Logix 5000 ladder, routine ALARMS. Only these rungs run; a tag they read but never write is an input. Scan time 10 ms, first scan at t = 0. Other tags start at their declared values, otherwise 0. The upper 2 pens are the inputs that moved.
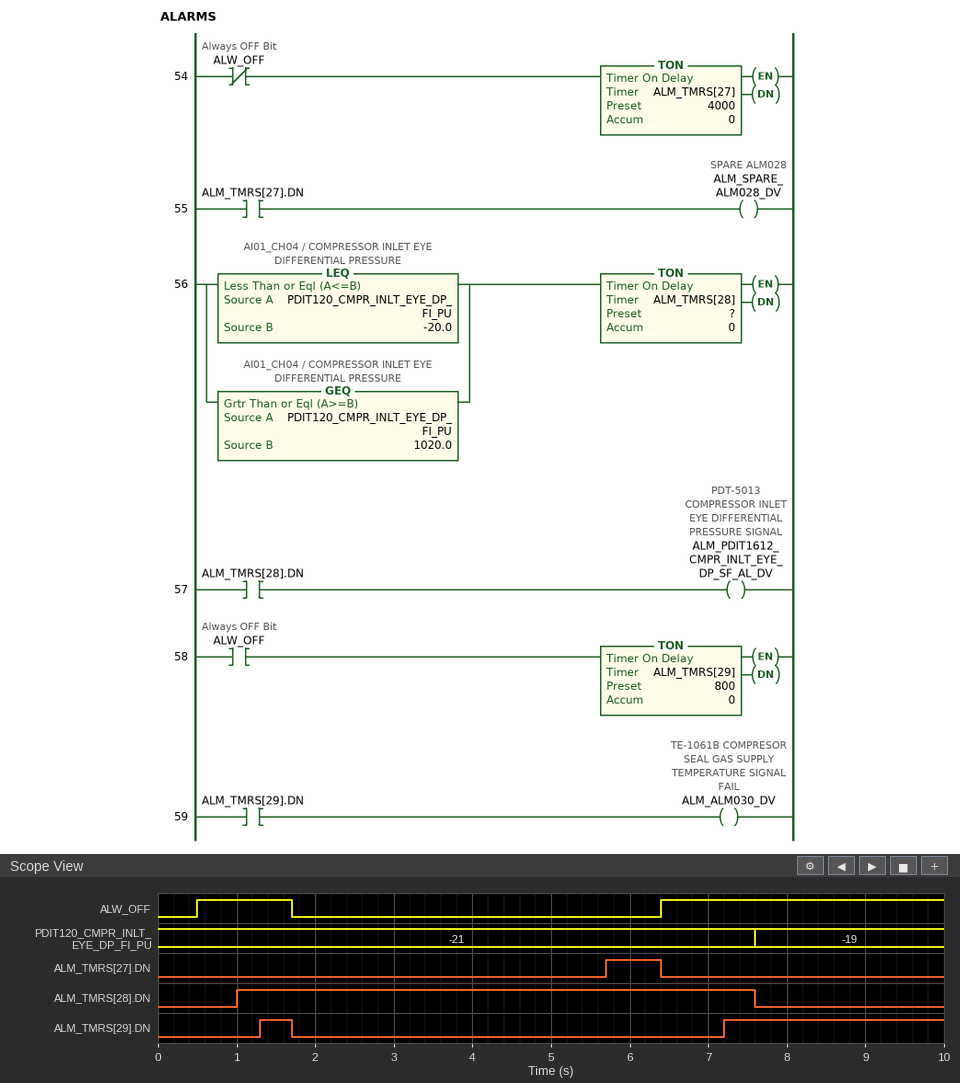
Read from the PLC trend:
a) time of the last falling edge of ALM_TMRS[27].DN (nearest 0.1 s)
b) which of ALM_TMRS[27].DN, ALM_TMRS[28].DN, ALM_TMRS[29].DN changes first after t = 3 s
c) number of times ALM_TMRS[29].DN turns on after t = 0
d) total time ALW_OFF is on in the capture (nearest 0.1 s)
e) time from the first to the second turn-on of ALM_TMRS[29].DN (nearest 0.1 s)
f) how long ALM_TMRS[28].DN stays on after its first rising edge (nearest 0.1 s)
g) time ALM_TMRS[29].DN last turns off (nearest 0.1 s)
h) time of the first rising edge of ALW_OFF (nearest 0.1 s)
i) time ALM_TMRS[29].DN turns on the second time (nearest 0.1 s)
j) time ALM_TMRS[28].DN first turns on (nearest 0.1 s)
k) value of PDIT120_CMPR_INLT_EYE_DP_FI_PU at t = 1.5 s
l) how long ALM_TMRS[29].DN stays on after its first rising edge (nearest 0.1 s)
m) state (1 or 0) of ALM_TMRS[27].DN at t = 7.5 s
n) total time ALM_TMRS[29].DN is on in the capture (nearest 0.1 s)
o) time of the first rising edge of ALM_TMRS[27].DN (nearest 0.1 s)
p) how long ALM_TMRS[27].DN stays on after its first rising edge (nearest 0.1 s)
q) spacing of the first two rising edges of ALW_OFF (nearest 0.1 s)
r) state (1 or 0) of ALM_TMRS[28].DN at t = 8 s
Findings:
6.4 s
ALM_TMRS[27].DN
2
4.8 s
5.9 s
6.6 s
1.7 s
0.5 s
7.2 s
1.0 s
-21
0.4 s
0
3.2 s
5.7 s
0.7 s
5.9 s
0
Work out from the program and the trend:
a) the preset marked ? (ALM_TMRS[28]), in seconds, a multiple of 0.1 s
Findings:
1.0 s
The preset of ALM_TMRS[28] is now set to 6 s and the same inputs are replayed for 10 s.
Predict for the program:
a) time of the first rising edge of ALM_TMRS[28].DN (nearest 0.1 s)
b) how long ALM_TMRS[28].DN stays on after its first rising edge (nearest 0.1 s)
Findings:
6.0 s
1.6 s
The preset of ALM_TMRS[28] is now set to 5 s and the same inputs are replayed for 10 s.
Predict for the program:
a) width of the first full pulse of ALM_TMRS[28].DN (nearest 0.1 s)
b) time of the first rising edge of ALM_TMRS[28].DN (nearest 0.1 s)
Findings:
2.6 s
5.0 s
